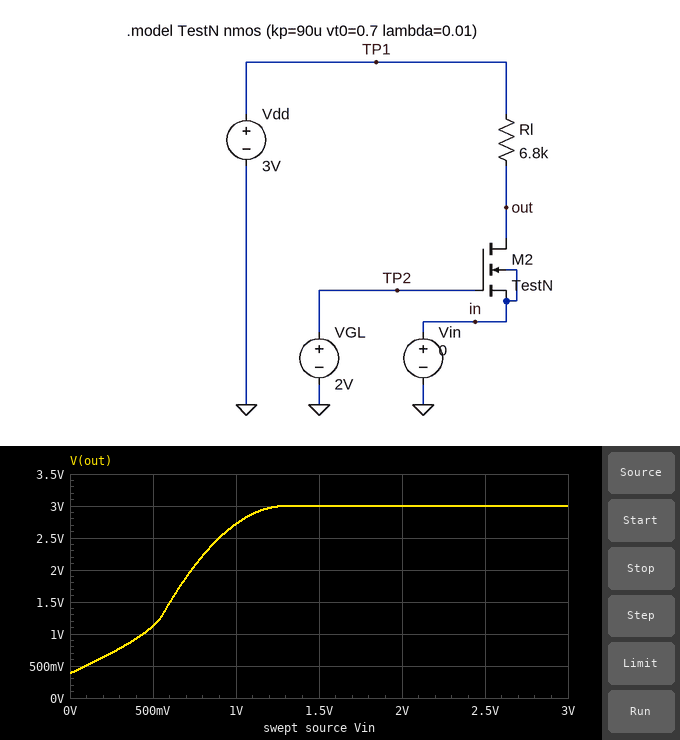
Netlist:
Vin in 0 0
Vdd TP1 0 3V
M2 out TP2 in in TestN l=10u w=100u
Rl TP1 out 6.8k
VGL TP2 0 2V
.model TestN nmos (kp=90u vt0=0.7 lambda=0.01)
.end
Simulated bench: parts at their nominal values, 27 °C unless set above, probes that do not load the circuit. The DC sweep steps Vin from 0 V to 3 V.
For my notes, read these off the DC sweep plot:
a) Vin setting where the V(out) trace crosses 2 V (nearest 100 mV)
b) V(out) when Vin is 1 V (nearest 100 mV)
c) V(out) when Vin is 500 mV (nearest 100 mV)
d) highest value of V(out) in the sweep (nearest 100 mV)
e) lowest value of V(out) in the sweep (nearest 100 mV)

700 mV
2.7 V
1.1 V
3.0 V
400 mV
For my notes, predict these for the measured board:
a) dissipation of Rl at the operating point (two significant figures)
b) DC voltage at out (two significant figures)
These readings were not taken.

1.0 mW
380 mV
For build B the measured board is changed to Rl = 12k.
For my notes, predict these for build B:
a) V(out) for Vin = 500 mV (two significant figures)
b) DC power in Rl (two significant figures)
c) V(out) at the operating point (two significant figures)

810 mV
650 µW
220 mV
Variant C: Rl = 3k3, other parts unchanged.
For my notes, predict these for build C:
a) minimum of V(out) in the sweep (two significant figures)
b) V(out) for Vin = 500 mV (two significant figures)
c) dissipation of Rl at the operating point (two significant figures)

820 mV
2.0 V
1.4 mW
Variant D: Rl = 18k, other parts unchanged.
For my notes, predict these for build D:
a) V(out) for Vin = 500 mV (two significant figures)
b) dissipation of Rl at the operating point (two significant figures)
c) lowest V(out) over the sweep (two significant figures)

700 mV
450 µW
140 mV
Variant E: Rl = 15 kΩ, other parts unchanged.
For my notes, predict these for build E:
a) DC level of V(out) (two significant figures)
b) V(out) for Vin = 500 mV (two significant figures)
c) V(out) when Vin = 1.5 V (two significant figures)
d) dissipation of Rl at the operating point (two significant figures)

170 mV
750 mV
3.0 V
530 µW
